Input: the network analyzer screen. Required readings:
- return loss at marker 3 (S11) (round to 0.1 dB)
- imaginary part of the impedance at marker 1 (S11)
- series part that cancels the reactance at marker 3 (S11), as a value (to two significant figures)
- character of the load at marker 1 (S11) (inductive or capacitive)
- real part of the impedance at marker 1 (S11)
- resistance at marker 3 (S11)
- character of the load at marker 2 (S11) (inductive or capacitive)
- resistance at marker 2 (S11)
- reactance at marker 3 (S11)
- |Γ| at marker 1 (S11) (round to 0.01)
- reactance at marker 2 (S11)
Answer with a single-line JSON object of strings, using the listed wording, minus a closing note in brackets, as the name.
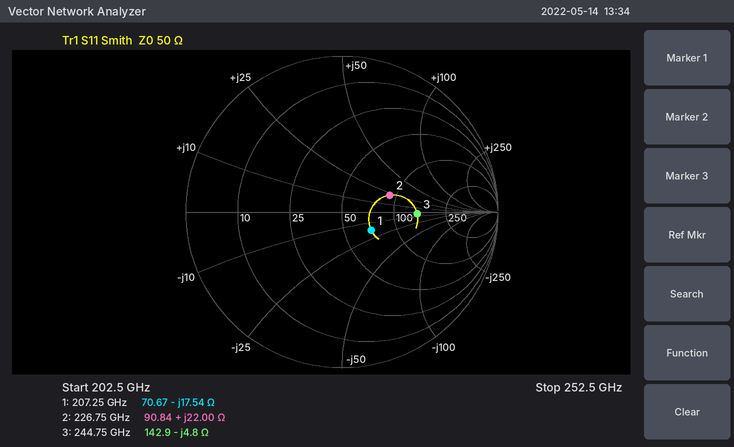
{"return loss at marker 3 (S11)": "6.3 dB", "imaginary part of the impedance at marker 1": "-17.54 Ω", "series part that cancels the reactance at marker 3 (S11), as a value": "3.1 pH", "character of the load at marker 1 (S11)": "capacitive", "real part of the impedance at marker 1": "70.67 Ω", "resistance at marker 3": "142.9 Ω", "character of the load at marker 2 (S11)": "inductive", "resistance at marker 2": "90.84 Ω", "reactance at marker 3": "-4.8 Ω", "|Γ| at marker 1 (S11)": "0.22", "reactance at marker 2": "+22.00 Ω"}
